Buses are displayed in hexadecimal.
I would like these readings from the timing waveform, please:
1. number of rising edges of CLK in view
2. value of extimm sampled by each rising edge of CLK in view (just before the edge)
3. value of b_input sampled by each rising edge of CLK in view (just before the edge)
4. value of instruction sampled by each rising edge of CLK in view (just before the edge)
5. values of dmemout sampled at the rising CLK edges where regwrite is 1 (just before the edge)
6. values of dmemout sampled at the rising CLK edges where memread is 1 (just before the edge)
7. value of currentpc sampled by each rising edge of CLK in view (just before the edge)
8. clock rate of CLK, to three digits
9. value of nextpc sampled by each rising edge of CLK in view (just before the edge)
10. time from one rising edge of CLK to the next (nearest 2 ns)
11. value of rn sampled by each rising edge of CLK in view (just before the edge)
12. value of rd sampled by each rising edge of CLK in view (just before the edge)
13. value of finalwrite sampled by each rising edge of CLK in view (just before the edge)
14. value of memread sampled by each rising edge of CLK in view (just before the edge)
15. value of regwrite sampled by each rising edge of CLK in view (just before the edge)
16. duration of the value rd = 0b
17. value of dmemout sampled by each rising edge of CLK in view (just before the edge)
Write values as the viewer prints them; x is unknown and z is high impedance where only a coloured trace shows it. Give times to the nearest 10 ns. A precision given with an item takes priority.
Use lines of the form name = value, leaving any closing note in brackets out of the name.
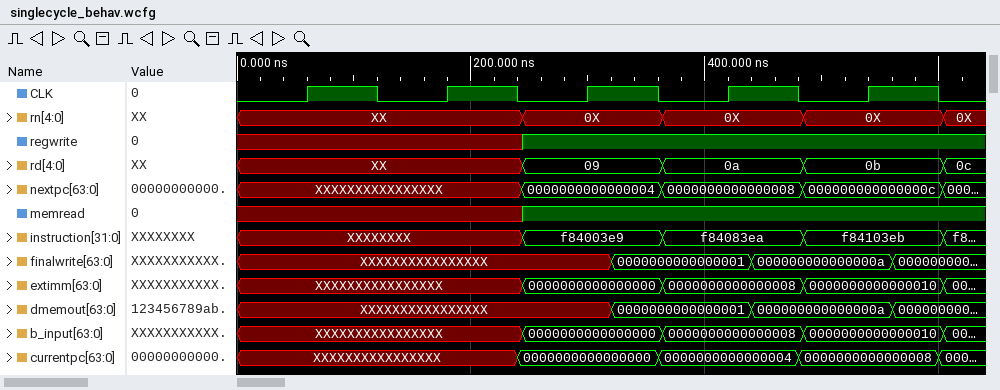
number of rising edges of CLK in view = 5
value of extimm sampled by each rising edge of CLK in view = XXXXXXXXXXXXXXXX, XXXXXXXXXXXXXXXX, 0000000000000000, 0000000000000008, 0000000000000010
value of b_input sampled by each rising edge of CLK in view = XXXXXXXXXXXXXXXX, XXXXXXXXXXXXXXXX, 0000000000000000, 0000000000000008, 0000000000000010
value of instruction sampled by each rising edge of CLK in view = XXXXXXXX, XXXXXXXX, f84003e9, f84083ea, f84103eb
values of dmemout sampled at the rising CLK edges where regwrite is 1 = XXXXXXXXXXXXXXXX, 0000000000000001, 000000000000000a
values of dmemout sampled at the rising CLK edges where memread is 1 = XXXXXXXXXXXXXXXX, 0000000000000001, 000000000000000a
value of currentpc sampled by each rising edge of CLK in view = XXXXXXXXXXXXXXXX, XXXXXXXXXXXXXXXX, 0000000000000000, 0000000000000004, 0000000000000008
clock rate of CLK, to three digits = 8.33 MHz
value of nextpc sampled by each rising edge of CLK in view = XXXXXXXXXXXXXXXX, XXXXXXXXXXXXXXXX, 0000000000000004, 0000000000000008, 000000000000000c
time from one rising edge of CLK to the next = 120 ns
value of rn sampled by each rising edge of CLK in view = XX, XX, 0X, 0X, 0X
value of rd sampled by each rising edge of CLK in view = XX, XX, 09, 0a, 0b
value of finalwrite sampled by each rising edge of CLK in view = XXXXXXXXXXXXXXXX, XXXXXXXXXXXXXXXX, XXXXXXXXXXXXXXXX, 0000000000000001, 000000000000000a
value of memread sampled by each rising edge of CLK in view = x x 1 1 1
value of regwrite sampled by each rising edge of CLK in view = x x 1 1 1
duration of the value rd = 0b = 120 ns
value of dmemout sampled by each rising edge of CLK in view = XXXXXXXXXXXXXXXX, XXXXXXXXXXXXXXXX, XXXXXXXXXXXXXXXX, 0000000000000001, 000000000000000a
